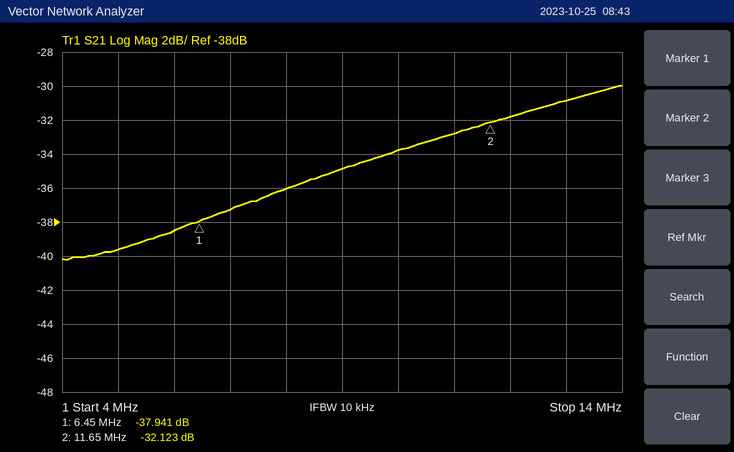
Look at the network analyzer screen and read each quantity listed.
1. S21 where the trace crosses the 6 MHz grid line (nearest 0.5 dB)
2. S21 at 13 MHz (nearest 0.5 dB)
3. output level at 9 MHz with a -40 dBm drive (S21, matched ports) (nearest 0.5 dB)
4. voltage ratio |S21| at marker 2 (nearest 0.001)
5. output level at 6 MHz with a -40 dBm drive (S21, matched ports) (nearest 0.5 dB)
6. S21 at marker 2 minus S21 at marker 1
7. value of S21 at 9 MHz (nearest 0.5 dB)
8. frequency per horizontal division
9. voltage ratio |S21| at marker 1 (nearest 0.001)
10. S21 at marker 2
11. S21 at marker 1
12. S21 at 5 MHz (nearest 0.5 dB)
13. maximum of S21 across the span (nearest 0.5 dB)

-38.5 dB
-31.0 dB
-75.0 dBm
0.025
-78.5 dBm
5.818 dB
-35.0 dB
1 MHz
0.013
-32.123 dB
-37.941 dB
-39.5 dB
-30.0 dB
